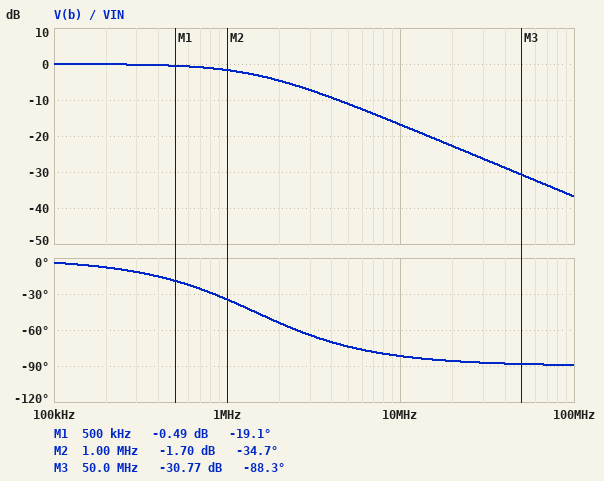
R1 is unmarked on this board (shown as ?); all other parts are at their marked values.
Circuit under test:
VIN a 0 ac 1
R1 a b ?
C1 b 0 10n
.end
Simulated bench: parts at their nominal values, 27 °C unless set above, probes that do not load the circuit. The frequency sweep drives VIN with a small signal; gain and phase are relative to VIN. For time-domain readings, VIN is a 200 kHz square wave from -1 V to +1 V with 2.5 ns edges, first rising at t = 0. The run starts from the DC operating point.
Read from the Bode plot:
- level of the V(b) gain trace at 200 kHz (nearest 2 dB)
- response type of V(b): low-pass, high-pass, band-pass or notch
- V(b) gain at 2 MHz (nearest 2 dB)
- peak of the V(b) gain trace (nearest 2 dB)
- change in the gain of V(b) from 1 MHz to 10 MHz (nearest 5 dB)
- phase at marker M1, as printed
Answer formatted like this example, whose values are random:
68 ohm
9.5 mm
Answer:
0 dB
low-pass
-4 dB
0 dB
-15 dB
-19.1 deg
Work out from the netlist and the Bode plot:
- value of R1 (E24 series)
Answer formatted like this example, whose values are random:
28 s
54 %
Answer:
11 Ω
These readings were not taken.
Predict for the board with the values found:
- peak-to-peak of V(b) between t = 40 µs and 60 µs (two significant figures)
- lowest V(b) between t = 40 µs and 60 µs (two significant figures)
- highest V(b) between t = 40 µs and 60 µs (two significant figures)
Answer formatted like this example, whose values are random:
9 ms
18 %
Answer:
2.0 V
-1.0 V
1.0 V
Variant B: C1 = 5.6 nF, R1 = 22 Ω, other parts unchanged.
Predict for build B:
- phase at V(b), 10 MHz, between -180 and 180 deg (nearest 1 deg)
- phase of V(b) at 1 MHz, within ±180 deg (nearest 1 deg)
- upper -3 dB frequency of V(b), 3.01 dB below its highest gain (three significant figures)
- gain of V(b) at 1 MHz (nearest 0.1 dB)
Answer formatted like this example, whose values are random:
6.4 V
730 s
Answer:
-83 deg
-38 deg
1.29 MHz
-2.0 dB
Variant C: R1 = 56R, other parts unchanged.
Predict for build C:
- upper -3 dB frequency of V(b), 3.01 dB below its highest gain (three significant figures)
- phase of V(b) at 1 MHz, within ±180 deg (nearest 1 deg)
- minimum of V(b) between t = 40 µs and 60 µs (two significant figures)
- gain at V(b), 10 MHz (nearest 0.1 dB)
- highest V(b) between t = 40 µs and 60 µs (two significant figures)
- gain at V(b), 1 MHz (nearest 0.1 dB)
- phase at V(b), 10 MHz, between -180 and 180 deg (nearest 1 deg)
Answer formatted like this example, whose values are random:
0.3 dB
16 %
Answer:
284 kHz
-74 deg
-980 mV
-30.9 dB
980 mV
-11.3 dB
-88 deg
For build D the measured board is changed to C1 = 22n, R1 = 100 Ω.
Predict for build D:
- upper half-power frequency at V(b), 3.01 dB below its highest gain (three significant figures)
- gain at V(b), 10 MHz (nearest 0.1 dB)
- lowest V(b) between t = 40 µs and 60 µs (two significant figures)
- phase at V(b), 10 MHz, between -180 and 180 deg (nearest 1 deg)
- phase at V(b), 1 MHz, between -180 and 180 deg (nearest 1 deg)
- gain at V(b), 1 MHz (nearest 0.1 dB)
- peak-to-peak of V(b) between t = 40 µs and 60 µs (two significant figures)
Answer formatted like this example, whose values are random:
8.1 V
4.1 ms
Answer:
72.3 kHz
-42.8 dB
-510 mV
-90 deg
-86 deg
-22.8 dB
1.0 V
